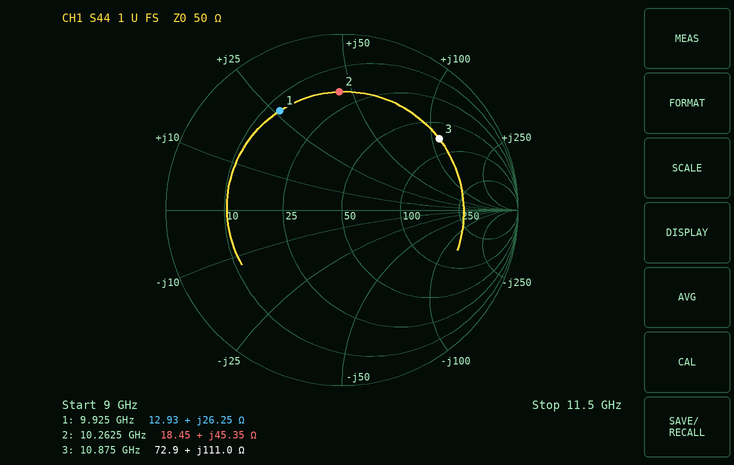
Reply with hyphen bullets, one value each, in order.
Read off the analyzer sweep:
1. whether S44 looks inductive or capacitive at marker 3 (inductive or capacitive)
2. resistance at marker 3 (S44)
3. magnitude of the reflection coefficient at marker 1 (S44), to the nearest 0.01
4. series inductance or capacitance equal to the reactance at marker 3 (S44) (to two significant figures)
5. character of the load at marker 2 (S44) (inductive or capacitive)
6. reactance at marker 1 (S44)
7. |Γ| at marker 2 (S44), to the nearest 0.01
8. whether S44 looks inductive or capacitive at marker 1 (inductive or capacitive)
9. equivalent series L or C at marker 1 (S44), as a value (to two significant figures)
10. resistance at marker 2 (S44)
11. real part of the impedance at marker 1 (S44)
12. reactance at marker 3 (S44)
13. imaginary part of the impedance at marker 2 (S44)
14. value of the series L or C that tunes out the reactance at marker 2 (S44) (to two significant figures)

- inductive
- 72.9 Ω
- 0.67
- 1.6 nH
- inductive
- +26.25 Ω
- 0.67
- inductive
- 420 pH
- 18.45 Ω
- 12.93 Ω
- +111.0 Ω
- +45.35 Ω
- 340 fF
